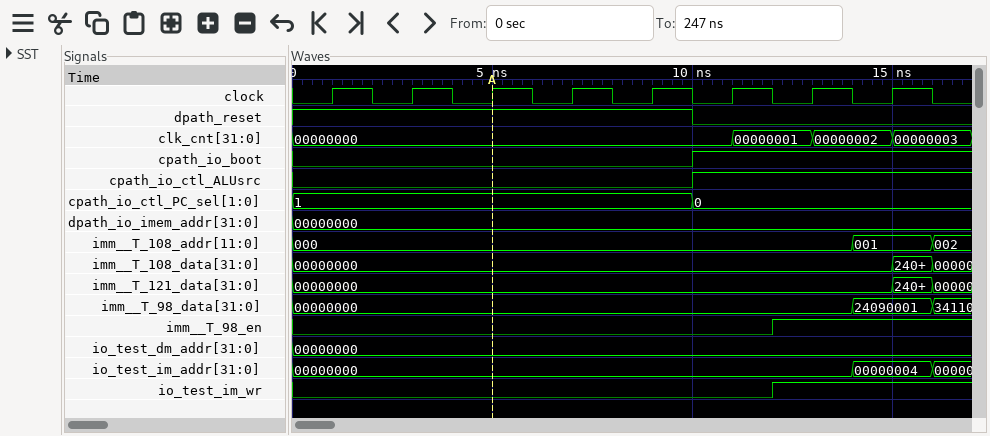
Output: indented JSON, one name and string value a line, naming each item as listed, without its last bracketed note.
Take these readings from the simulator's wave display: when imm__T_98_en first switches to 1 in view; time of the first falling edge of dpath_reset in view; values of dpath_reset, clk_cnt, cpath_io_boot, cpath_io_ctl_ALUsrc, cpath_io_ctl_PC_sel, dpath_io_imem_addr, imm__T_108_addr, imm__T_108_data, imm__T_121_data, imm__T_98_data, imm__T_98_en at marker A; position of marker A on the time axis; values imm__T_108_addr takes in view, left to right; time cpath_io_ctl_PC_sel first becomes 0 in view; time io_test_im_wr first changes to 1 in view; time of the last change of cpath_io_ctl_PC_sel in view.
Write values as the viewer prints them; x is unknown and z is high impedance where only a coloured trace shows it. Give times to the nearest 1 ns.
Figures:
{
  "when imm__T_98_en first switches to 1 in view": "12 ns",
  "time of the first falling edge of dpath_reset in view": "10 ns",
  "values of dpath_reset, clk_cnt, cpath_io_boot, cpath_io_ctl_ALUsrc, cpath_io_ctl_PC_sel, dpath_io_imem_addr, imm__T_108_addr, imm__T_108_data, imm__T_121_data, imm__T_98_data, imm__T_98_en at marker A": "dpath_reset=1, clk_cnt=00000000, cpath_io_boot=0, cpath_io_ctl_ALUsrc=0, cpath_io_ctl_PC_sel=1, dpath_io_imem_addr=00000000, imm__T_108_addr=000, imm__T_108_data=00000000, imm__T_121_data=00000000, imm__T_98_data=00000000, imm__T_98_en=0",
  "position of marker A on the time axis": "5 ns",
  "values imm__T_108_addr takes in view, left to right": "000, 001, 002",
  "time cpath_io_ctl_PC_sel first becomes 0 in view": "10 ns",
  "time io_test_im_wr first changes to 1 in view": "12 ns",
  "time of the last change of cpath_io_ctl_PC_sel in view": "10 ns"
}
